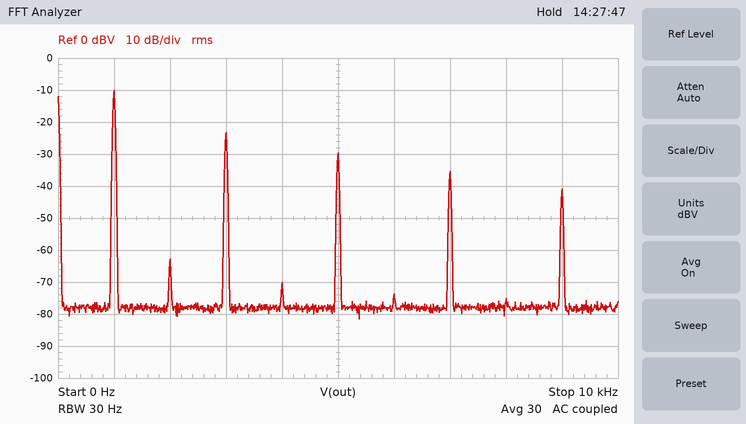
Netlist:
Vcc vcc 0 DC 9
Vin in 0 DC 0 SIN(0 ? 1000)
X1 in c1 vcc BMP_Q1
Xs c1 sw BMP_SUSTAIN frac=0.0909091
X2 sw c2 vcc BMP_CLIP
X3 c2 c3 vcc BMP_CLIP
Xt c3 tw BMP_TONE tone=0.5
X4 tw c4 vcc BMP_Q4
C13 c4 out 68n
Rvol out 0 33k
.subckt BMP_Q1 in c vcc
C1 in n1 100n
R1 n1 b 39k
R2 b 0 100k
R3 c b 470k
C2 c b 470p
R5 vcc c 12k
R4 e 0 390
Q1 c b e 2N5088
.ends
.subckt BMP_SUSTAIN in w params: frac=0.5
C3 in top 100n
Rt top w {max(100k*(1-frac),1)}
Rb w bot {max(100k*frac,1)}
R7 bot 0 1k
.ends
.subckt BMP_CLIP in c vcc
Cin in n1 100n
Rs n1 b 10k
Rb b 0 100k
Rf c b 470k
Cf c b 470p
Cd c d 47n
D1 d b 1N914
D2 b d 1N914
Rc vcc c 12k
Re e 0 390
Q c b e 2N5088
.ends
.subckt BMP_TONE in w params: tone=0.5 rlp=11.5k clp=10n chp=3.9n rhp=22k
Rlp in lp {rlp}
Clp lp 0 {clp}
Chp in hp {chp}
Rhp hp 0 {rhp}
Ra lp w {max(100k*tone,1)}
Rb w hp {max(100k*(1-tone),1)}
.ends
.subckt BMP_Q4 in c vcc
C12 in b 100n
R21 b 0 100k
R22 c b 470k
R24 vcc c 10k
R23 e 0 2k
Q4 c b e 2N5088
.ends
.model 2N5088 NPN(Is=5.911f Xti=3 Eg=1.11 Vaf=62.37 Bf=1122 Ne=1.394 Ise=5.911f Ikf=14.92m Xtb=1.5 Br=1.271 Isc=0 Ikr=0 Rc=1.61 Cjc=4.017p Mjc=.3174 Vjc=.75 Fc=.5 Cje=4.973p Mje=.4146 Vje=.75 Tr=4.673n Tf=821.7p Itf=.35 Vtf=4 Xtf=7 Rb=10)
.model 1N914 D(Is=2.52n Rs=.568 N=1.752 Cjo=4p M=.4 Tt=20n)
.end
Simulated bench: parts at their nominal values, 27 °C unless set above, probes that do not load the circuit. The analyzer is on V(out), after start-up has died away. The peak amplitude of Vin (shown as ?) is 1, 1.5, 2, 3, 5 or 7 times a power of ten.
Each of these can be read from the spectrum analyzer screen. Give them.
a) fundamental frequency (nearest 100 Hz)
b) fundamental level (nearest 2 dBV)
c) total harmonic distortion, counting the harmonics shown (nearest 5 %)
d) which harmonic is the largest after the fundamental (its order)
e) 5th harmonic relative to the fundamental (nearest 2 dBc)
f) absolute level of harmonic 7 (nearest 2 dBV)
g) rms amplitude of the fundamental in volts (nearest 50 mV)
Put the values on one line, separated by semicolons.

1.0 kHz; -10 dBV; 25 %; 3; -20 dBc; -36 dBV; 300 mV
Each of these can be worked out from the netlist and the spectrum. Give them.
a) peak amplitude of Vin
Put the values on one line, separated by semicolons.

70 mV
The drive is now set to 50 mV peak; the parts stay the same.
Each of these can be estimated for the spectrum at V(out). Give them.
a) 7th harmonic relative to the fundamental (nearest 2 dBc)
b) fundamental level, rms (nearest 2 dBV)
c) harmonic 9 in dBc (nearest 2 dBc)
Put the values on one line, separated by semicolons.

-28 dBc; -10 dBV; -34 dBc
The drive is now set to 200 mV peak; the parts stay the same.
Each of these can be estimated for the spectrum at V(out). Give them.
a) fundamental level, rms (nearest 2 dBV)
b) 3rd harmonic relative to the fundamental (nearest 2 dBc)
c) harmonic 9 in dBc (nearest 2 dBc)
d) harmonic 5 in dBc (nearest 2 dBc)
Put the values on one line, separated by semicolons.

-10 dBV; -12 dBc; -24 dBc; -16 dBc
